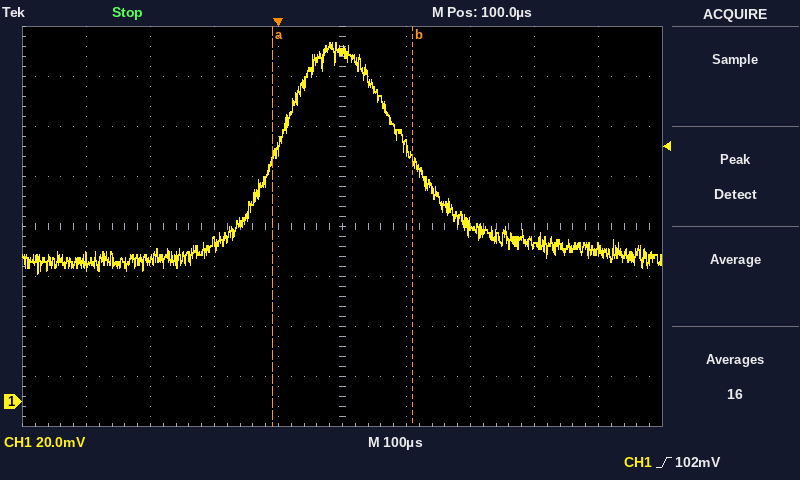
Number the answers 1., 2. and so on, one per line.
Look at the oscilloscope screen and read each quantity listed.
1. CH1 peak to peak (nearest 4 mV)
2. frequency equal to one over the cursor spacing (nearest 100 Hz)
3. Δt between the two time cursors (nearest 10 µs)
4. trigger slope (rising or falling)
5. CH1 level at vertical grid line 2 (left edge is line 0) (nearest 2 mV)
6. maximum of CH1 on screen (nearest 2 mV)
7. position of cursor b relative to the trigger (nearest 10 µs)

1. 92 mV
2. 4.5 kHz
3. 220 µs
4. rising
5. 56 mV
6. 144 mV
7. +210 µs
